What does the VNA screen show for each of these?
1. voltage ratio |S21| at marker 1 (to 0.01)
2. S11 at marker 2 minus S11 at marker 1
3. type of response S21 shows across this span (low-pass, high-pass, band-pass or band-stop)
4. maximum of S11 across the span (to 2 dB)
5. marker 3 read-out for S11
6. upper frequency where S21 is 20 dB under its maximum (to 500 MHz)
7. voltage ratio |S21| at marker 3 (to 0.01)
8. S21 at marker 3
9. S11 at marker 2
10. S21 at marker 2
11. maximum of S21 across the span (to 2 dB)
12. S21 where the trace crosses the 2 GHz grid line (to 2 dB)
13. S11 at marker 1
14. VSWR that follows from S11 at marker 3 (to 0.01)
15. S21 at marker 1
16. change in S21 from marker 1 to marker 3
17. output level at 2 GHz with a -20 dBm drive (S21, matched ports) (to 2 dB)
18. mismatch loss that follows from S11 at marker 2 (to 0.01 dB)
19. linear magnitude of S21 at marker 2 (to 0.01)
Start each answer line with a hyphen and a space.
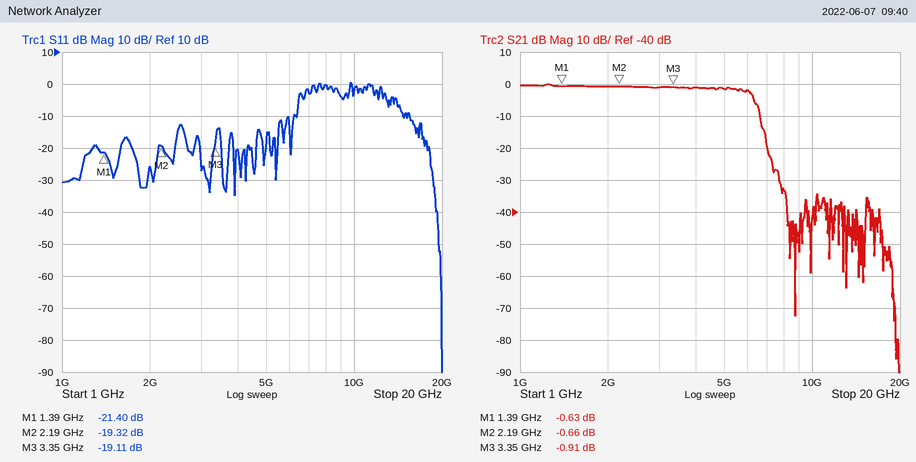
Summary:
- 0.93
- 2.08 dB
- low-pass
- 0 dB
- -19.11 dB
- 7.0 GHz
- 0.90
- -0.91 dB
- -19.32 dB
- -0.66 dB
- 0 dB
- 0 dB
- -21.40 dB
- 1.25
- -0.63 dB
- -0.28 dB
- -20 dBm
- 0.05 dB
- 0.93
